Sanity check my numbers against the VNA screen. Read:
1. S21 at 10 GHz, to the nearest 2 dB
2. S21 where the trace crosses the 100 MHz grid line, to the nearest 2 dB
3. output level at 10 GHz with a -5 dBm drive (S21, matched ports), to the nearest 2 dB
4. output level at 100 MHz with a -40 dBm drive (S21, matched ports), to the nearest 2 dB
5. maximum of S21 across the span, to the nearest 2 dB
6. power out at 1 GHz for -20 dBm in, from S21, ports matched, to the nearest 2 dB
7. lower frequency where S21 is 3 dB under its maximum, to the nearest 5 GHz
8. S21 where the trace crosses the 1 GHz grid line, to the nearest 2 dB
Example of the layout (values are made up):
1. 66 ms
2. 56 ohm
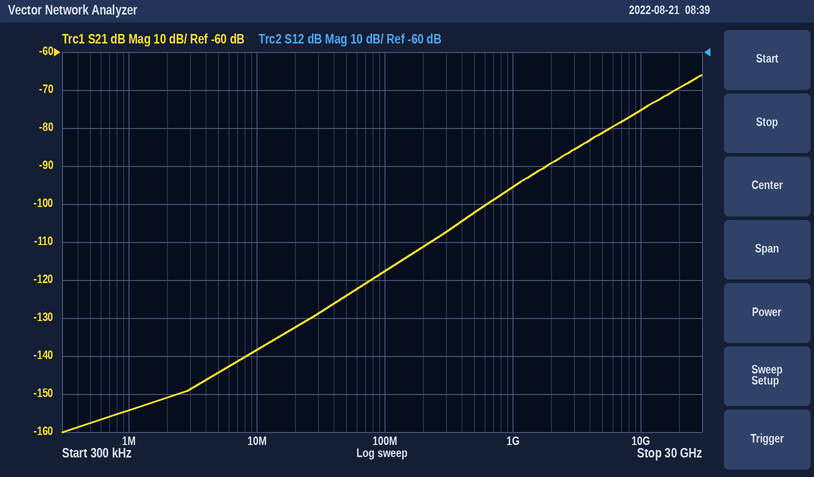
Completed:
1. -76 dB
2. -118 dB
3. -80 dBm
4. -158 dBm
5. -66 dB
6. -116 dBm
7. 20 GHz
8. -96 dB
